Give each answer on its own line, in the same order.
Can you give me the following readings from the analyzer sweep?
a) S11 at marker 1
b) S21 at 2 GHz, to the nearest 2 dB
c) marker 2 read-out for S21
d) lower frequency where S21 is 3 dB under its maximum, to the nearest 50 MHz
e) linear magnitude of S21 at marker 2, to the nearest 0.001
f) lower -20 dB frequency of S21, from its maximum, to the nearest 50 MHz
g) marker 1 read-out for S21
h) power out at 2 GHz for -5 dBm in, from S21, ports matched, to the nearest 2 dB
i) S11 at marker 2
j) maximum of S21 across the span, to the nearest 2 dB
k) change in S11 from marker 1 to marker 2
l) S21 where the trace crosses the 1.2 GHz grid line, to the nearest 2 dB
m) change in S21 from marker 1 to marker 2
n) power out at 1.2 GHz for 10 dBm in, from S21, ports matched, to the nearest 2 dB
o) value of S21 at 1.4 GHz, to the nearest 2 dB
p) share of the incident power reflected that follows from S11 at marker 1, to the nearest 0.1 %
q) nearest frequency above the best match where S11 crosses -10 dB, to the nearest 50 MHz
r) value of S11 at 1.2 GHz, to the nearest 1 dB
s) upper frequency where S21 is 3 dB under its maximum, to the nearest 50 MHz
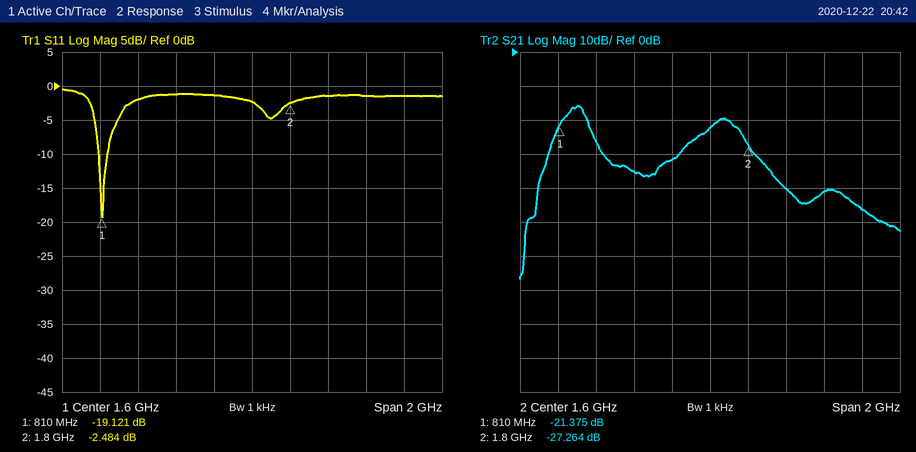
-19.121 dB
-40 dB
-27.264 dB
850 MHz
0.043
700 MHz
-21.375 dB
-46 dBm
-2.484 dB
-16 dB
16.637 dB
-36 dB
-5.889 dB
-26 dBm
-32 dB
1.2 %
850 MHz
-1 dB
950 MHz
